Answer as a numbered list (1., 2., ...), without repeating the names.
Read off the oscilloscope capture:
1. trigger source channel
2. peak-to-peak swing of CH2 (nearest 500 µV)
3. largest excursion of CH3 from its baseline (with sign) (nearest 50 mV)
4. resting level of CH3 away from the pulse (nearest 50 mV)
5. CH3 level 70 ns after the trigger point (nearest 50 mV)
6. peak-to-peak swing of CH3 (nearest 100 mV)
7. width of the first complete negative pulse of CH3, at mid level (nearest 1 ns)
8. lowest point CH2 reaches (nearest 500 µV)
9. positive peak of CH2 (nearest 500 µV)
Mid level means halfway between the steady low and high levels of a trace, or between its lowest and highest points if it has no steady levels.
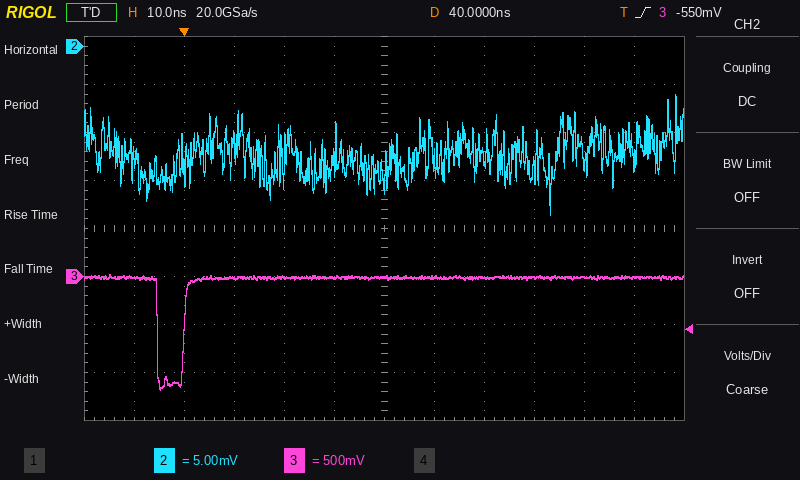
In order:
1. CH3
2. 12.5 mV
3. -1.15 V
4. 0 mV
5. 0 mV
6. 1.20 V
7. 5 ns
8. -17.5 mV
9. -5.0 mV
